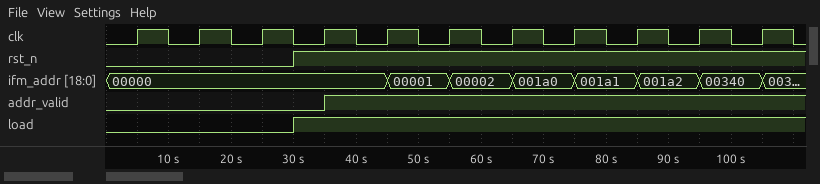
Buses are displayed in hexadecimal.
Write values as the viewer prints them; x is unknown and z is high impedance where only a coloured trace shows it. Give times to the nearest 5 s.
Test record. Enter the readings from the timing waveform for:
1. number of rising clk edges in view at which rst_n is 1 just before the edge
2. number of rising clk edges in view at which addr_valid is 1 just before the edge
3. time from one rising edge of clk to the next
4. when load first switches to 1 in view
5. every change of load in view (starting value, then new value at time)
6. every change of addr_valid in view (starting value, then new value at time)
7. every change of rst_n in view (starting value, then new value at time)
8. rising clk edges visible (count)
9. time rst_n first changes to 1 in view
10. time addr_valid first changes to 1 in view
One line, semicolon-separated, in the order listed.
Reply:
8; 7; 10 s; 30 s; 0, 1 at 30 s; 0, 1 at 35 s; 0, 1 at 30 s; 11; 30 s; 35 s
